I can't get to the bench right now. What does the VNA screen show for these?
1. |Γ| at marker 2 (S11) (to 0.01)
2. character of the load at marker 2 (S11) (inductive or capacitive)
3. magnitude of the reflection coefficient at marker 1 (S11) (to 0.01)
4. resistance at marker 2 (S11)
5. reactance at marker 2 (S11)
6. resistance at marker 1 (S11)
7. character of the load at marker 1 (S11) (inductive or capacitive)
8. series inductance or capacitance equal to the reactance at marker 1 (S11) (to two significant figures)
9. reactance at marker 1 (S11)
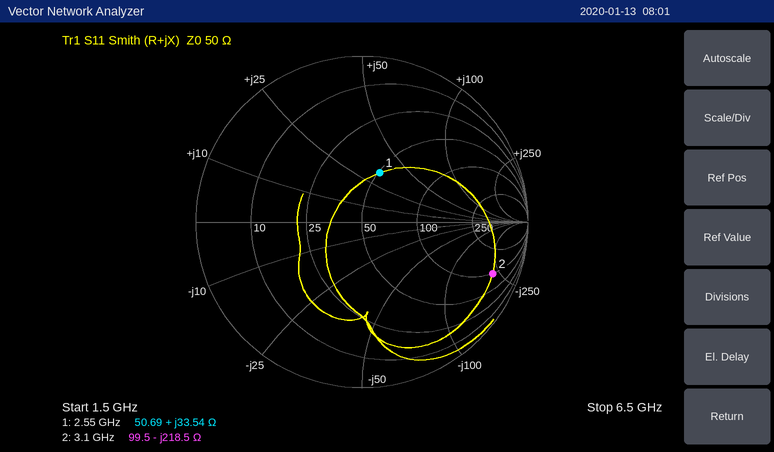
0.85
capacitive
0.32
99.5 Ω
-218.5 Ω
50.69 Ω
inductive
2.1 nH
+33.54 Ω
